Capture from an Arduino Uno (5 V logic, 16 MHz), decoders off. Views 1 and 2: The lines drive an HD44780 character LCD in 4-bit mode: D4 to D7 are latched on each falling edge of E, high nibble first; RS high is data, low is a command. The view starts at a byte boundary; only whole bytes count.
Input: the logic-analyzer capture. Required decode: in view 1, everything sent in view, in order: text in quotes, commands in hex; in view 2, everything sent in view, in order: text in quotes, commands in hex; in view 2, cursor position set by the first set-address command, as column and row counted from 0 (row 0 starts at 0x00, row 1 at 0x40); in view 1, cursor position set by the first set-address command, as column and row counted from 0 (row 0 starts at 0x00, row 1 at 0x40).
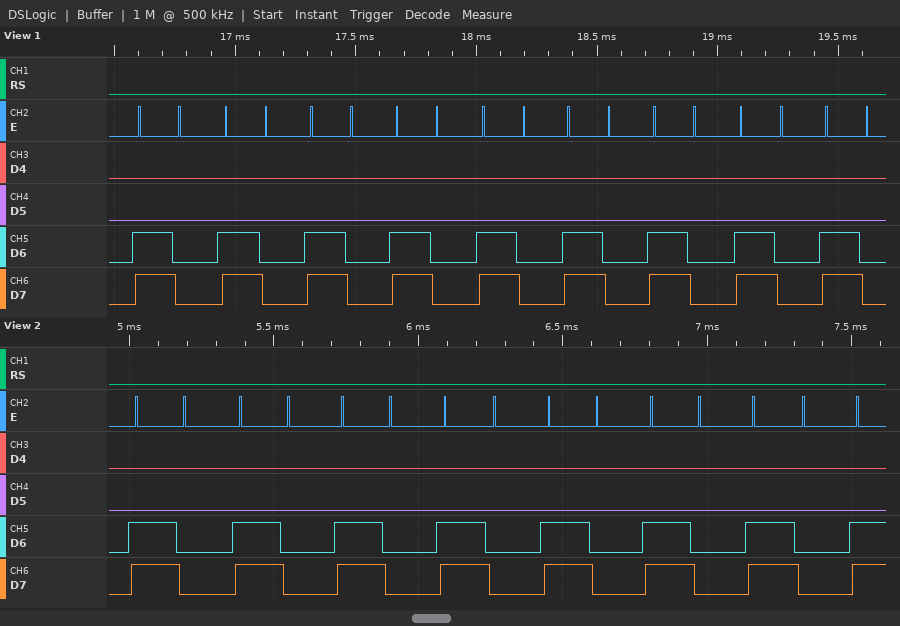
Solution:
0xC0 0xC0 0xC0 0xC0 0xC0 0xC0 0xC0 0xC0 0xC0
0xC0 0xC0 0xC0 0xC0 0xC0 0xC0 0xC0
column 0, row 1
column 0, row 1
